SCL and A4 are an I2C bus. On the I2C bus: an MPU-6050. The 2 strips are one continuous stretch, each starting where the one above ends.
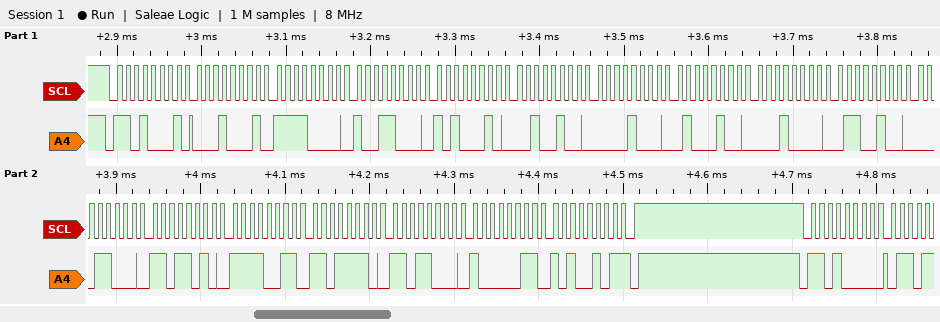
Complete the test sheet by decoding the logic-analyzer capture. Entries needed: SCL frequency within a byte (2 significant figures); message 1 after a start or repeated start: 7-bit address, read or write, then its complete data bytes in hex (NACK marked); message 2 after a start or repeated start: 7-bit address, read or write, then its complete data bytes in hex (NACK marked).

100 kHz
0x68 read: 11 F0 98 A2 24 08 44 10 64 18 DA F3 DE D8 83 A5 NACK
0x68 write
